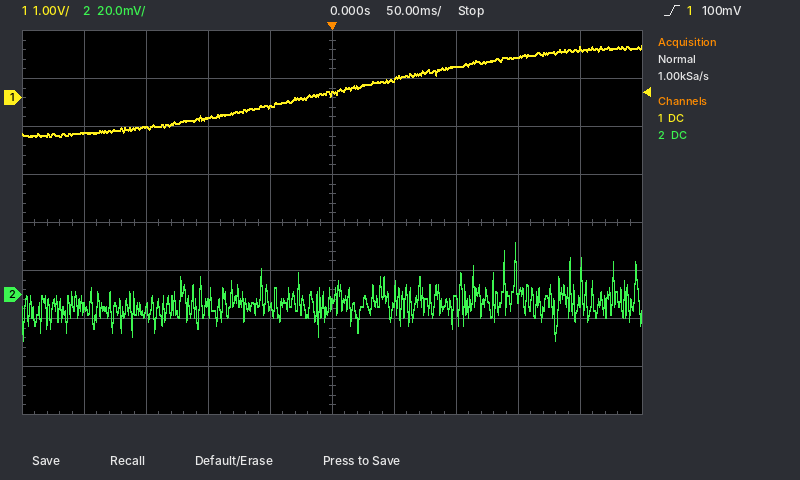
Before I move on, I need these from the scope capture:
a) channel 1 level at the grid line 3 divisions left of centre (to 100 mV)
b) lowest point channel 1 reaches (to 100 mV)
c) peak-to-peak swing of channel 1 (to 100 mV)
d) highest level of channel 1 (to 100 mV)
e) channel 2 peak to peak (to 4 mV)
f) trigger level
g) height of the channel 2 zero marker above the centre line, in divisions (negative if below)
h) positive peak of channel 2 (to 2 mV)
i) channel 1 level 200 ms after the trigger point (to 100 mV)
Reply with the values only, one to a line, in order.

-600 mV
-800 mV
1.9 V
1.1 V
40 mV
100 mV
-1.5 div
22 mV
1.0 V
